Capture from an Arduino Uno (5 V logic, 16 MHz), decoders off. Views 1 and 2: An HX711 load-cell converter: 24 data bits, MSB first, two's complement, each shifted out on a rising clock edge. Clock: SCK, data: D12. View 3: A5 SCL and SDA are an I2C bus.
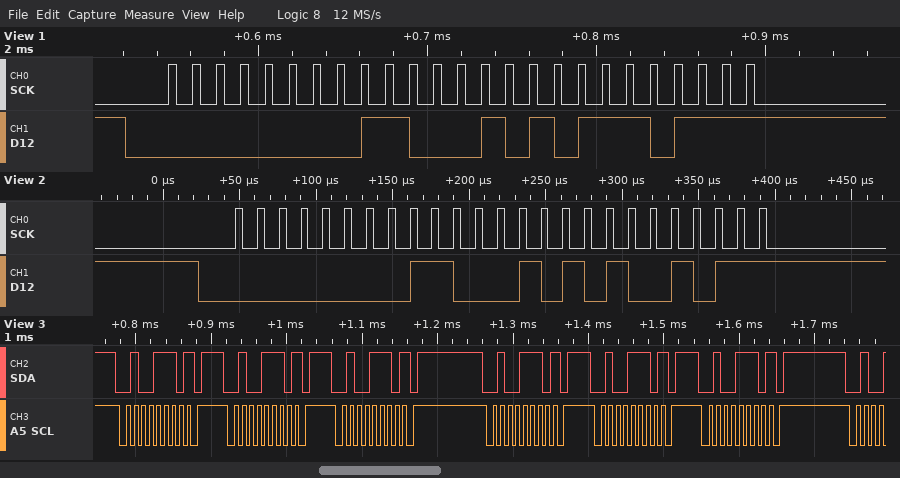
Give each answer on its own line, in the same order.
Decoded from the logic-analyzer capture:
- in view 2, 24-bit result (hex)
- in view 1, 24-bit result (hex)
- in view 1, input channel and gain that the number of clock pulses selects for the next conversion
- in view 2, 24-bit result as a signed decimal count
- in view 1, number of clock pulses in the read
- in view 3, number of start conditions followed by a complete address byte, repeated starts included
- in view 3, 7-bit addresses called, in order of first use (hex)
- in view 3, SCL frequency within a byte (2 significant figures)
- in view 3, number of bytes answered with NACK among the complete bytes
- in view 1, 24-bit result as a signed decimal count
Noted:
0x00C54B
0x00C577
channel A, gain 128
50507
25
6
0x27
100 kHz
6
50551
